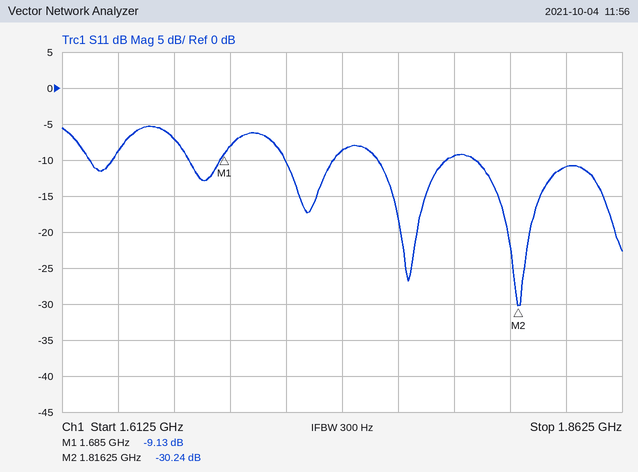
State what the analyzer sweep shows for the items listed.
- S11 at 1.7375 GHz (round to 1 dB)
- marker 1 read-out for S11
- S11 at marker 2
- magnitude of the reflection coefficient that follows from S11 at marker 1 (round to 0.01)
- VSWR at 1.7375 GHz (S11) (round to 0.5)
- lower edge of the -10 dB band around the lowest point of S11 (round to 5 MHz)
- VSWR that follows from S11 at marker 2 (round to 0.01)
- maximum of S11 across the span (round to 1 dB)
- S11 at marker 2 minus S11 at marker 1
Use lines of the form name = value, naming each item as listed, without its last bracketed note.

S11 at 1.7375 GHz = -9 dB
marker 1 read-out for S11 = -9.13 dB
S11 at marker 2 = -30.24 dB
magnitude of the reflection coefficient that follows from S11 at marker 1 = 0.35
VSWR at 1.7375 GHz (S11) = 2.0
lower edge of the -10 dB band around the lowest point of S11 = 1.795 GHz
VSWR that follows from S11 at marker 2 = 1.06
maximum of S11 across the span = -5 dB
S11 at marker 2 minus S11 at marker 1 = -21.11 dB
